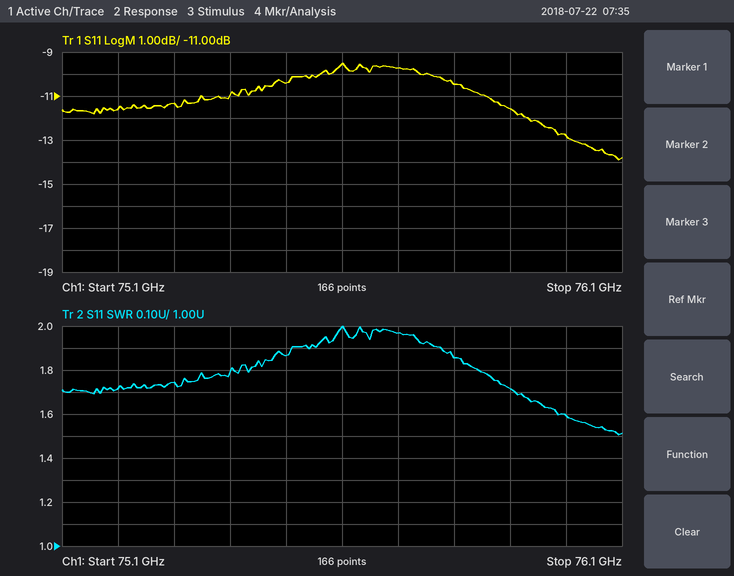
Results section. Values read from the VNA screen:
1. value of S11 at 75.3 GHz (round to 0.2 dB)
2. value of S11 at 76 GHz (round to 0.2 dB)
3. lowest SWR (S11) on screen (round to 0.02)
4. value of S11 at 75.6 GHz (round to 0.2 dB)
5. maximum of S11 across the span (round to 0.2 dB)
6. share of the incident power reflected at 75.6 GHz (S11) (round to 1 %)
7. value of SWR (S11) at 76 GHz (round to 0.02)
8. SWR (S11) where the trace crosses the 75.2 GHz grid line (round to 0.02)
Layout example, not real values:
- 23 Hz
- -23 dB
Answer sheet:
- -11.4 dB
- -12.8 dB
- 1.50
- -9.6 dB
- -9.6 dB
- 11 %
- 1.60
- 1.72
